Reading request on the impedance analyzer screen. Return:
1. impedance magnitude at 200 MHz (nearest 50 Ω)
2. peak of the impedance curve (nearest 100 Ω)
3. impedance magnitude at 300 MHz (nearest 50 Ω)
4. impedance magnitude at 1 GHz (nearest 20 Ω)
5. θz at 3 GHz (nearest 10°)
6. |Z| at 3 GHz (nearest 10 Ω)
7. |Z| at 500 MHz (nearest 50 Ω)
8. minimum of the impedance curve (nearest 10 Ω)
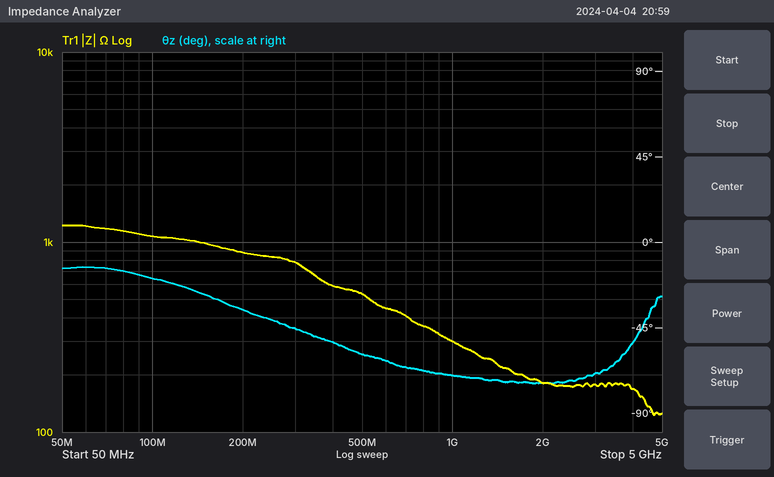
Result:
900 Ω
1.2 kΩ
800 Ω
300 Ω
-70°
180 Ω
550 Ω
120 Ω
